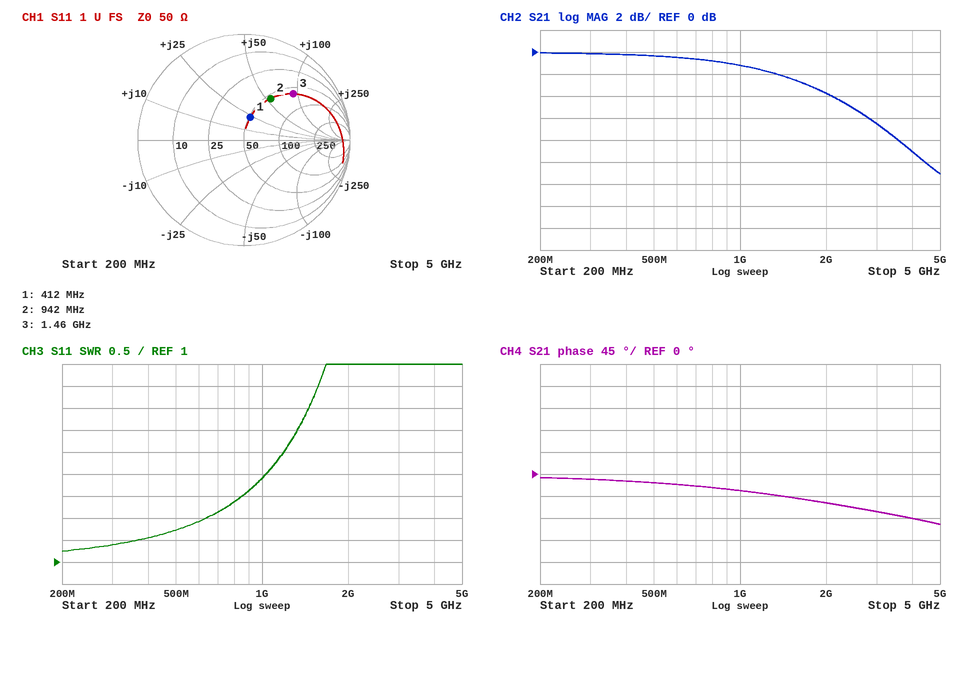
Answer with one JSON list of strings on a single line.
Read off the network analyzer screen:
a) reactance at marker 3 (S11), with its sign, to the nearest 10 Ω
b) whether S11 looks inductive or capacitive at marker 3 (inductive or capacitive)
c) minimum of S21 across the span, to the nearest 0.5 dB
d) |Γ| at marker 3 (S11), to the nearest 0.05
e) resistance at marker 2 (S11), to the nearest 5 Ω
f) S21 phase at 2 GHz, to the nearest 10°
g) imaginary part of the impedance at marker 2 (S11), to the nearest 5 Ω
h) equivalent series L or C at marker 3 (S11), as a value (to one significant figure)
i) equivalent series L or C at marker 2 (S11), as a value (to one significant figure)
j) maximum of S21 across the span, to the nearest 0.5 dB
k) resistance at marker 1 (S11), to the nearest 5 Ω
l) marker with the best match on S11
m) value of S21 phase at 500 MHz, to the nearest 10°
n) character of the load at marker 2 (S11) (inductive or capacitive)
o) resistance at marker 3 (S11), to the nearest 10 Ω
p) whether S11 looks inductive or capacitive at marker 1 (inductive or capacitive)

["+90 Ω", "inductive", "-11.0 dB", "0.65", "55 Ω", "-60°", "+55 Ω", "10 nH", "9 nH", "0.0 dB", "50 Ω", "marker 1", "-20°", "inductive", "60 Ω", "inductive"]
